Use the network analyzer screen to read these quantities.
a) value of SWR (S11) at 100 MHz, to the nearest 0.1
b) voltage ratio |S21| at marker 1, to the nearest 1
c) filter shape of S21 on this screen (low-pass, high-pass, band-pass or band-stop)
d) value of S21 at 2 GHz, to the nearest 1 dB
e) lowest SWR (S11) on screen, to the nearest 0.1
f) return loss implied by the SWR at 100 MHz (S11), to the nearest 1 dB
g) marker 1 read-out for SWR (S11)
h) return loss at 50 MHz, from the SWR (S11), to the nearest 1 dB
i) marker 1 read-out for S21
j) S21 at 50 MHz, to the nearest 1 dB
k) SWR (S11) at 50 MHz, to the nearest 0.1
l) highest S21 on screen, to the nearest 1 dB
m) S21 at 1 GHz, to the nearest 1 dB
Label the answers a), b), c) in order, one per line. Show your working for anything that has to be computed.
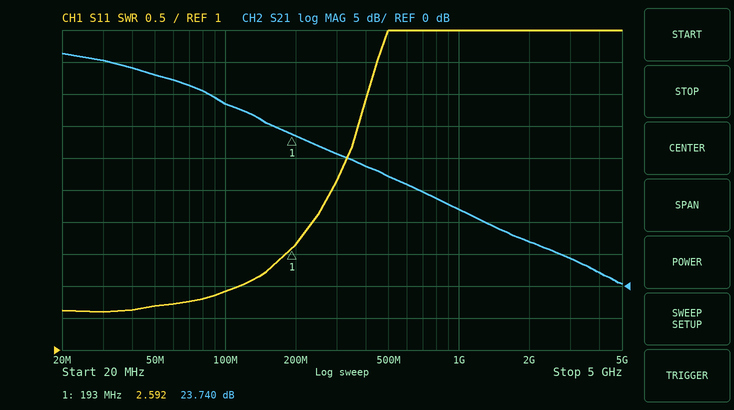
a) 1.9
b) 10^(23.74/20) ≈ 15
c) low-pass
d) 7 dB
e) 1.6
f) −20 log10((1.9 − 1)/(1.9 + 1)) ≈ 10 dB
g) 2.592
h) −20 log10((1.7 − 1)/(1.7 + 1)) ≈ 12 dB
i) 23.740 dB
j) 33 dB
k) 1.7
l) 36 dB
m) 12 dB
